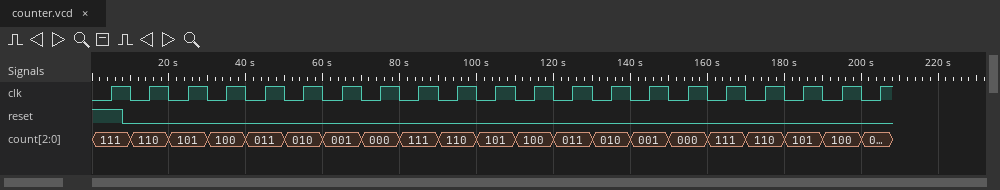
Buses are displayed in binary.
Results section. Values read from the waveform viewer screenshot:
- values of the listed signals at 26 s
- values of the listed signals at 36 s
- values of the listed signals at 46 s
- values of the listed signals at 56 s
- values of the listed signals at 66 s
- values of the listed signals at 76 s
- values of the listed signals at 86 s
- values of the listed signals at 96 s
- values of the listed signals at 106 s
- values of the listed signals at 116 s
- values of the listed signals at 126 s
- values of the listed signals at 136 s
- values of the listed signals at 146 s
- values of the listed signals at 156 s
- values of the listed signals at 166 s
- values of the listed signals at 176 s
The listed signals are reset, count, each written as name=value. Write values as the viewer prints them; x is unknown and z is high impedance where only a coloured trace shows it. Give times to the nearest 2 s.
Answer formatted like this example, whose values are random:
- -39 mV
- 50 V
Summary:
- reset=0, count=101
- reset=0, count=100
- reset=0, count=011
- reset=0, count=010
- reset=0, count=001
- reset=0, count=000
- reset=0, count=111
- reset=0, count=110
- reset=0, count=101
- reset=0, count=100
- reset=0, count=011
- reset=0, count=010
- reset=0, count=001
- reset=0, count=000
- reset=0, count=111
- reset=0, count=110
